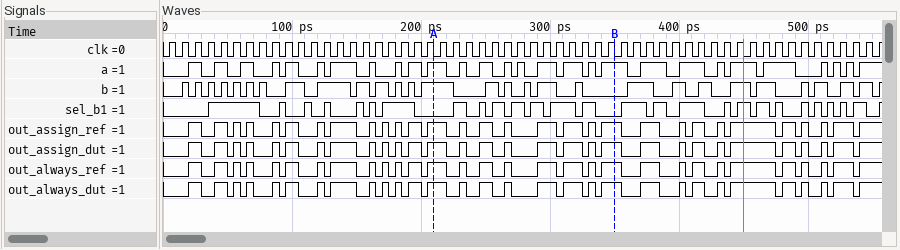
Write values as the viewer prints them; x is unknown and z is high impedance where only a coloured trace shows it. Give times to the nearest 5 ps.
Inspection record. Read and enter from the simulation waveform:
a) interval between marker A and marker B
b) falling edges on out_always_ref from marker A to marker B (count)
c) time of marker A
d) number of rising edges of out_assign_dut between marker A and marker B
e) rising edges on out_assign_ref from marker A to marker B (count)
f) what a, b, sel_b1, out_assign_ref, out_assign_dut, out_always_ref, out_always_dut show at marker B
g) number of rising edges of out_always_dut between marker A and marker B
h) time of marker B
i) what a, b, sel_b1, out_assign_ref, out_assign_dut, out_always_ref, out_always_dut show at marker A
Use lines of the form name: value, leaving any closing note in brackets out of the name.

interval between marker A and marker B: 140 ps
falling edges on out_always_ref from marker A to marker B: 7
time of marker A: 210 ps
number of rising edges of out_assign_dut between marker A and marker B: 7
rising edges on out_assign_ref from marker A to marker B: 7
what a, b, sel_b1, out_assign_ref, out_assign_dut, out_always_ref, out_always_dut show at marker B: a=1, b=0, sel_b1=0, out_assign_ref=1, out_assign_dut=1, out_always_ref=1, out_always_dut=1
number of rising edges of out_always_dut between marker A and marker B: 7
time of marker B: 350 ps
what a, b, sel_b1, out_assign_ref, out_assign_dut, out_always_ref, out_always_dut show at marker A: a=1, b=1, sel_b1=0, out_assign_ref=1, out_assign_dut=1, out_always_ref=1, out_always_dut=1
